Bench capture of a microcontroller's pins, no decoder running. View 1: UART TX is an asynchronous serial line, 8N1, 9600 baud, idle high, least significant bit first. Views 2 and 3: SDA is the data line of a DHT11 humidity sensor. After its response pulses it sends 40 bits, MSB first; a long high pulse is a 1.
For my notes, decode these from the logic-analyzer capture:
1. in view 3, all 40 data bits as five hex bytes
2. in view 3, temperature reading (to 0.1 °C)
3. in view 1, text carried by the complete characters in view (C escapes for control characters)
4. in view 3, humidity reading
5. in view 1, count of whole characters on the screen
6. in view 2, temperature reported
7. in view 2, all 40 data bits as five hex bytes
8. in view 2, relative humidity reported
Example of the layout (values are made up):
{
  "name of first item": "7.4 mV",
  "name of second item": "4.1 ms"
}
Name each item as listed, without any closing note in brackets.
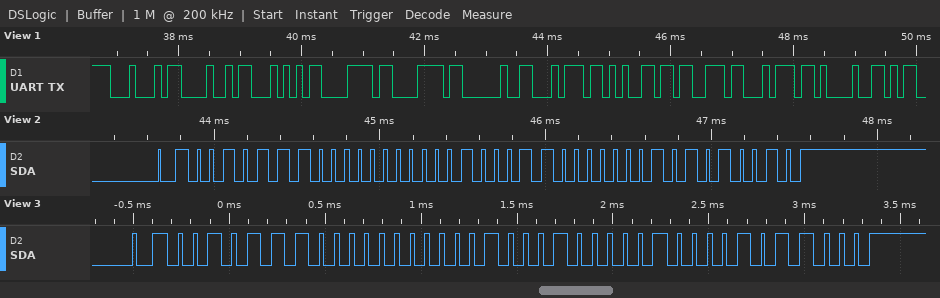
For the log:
{
  "in view 3, all 40 data bits as five hex bytes": "2E 00 22 08 58",
  "in view 3, temperature reading": "34.8 °C",
  "in view 1, text carried by the complete characters in view": "\"DHTxx test!\"",
  "in view 3, humidity reading": "46 %",
  "in view 1, count of whole characters on the screen": "11",
  "in view 2, temperature reported": "35.1 °C",
  "in view 2, all 40 data bits as five hex bytes": "2E 00 23 01 52",
  "in view 2, relative humidity reported": "46 %"
}
